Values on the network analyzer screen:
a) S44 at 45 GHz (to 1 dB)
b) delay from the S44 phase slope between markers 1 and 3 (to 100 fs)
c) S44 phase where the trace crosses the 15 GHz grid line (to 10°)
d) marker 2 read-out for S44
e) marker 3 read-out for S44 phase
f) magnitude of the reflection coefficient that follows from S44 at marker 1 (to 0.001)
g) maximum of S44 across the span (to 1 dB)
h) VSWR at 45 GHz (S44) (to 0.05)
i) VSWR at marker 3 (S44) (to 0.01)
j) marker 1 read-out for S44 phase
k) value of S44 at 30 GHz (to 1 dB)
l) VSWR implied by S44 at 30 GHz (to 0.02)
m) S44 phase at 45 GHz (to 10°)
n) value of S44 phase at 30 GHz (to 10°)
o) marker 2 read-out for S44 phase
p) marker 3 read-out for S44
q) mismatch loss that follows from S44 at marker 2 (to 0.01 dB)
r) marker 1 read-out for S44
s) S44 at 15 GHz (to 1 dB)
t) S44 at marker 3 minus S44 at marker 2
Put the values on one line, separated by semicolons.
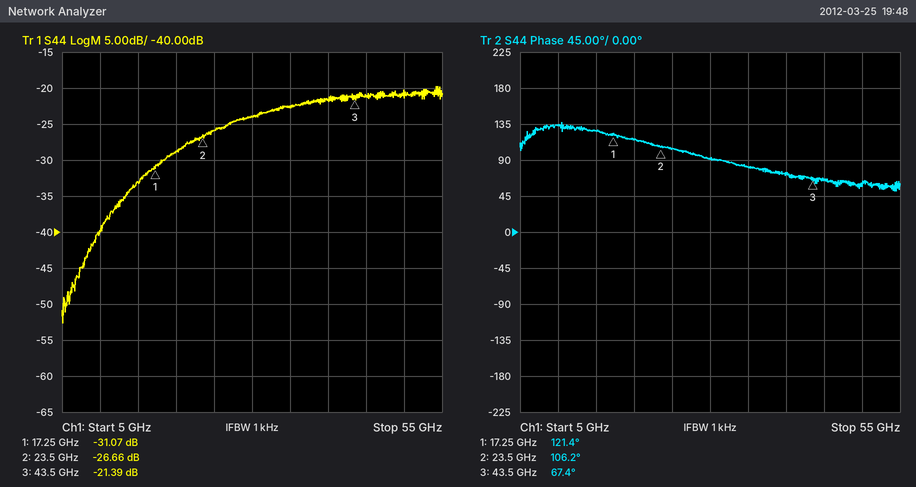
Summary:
-21 dB; 5.7 ps; 130°; -26.66 dB; 67.4°; 0.028; -20 dB; 1.20; 1.19; 121.4°; -24 dB; 1.14; 70°; 90°; 106.2°; -21.39 dB; 0.01 dB; -31.07 dB; -33 dB; 5.27 dB
